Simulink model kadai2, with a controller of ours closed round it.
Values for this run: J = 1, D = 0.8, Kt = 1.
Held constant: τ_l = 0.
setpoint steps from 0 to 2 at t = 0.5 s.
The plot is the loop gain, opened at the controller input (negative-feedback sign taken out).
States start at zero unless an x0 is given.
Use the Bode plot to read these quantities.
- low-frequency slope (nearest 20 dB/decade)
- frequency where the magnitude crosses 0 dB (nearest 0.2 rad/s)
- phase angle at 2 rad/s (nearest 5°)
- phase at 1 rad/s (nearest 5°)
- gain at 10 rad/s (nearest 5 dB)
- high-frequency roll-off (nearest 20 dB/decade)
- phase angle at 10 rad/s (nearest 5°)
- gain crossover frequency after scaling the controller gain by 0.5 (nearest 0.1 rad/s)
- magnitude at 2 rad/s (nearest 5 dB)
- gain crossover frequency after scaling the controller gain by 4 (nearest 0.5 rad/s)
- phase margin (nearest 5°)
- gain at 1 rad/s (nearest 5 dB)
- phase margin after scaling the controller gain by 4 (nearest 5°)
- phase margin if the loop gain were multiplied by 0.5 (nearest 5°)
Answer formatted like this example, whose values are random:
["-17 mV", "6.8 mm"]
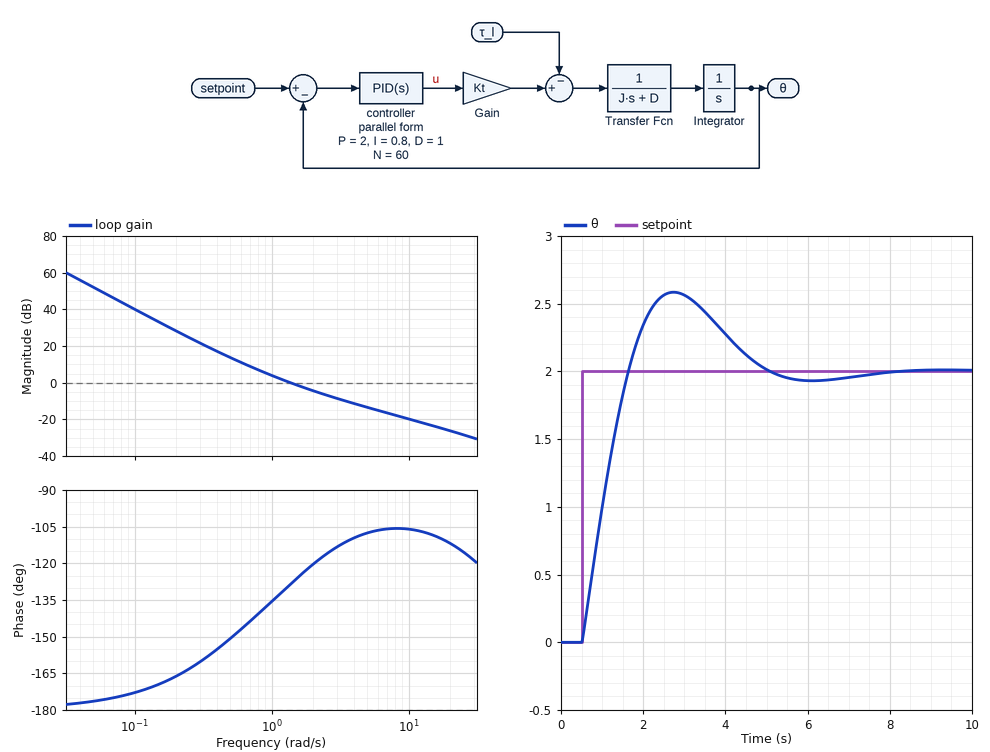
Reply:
["-40 dB/decade", "1.4 rad/s", "-120°", "-135°", "-20 dB", "-20 dB/decade", "-105°", "0.9 rad/s", "-5 dB", "4.5 rad/s", "50°", "5 dB", "70°", "40°"]
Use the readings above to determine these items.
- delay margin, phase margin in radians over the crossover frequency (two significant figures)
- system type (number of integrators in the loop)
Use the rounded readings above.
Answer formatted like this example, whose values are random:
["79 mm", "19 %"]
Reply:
["0.62 s", "2"]
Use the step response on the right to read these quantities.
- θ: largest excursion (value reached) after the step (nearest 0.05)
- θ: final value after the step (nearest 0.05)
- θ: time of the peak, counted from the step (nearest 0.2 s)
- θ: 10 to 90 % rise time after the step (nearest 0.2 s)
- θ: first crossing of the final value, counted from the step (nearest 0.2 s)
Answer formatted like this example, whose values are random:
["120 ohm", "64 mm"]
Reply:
["2.60", "2.00", "2.2 s", "0.8 s", "1.2 s"]
